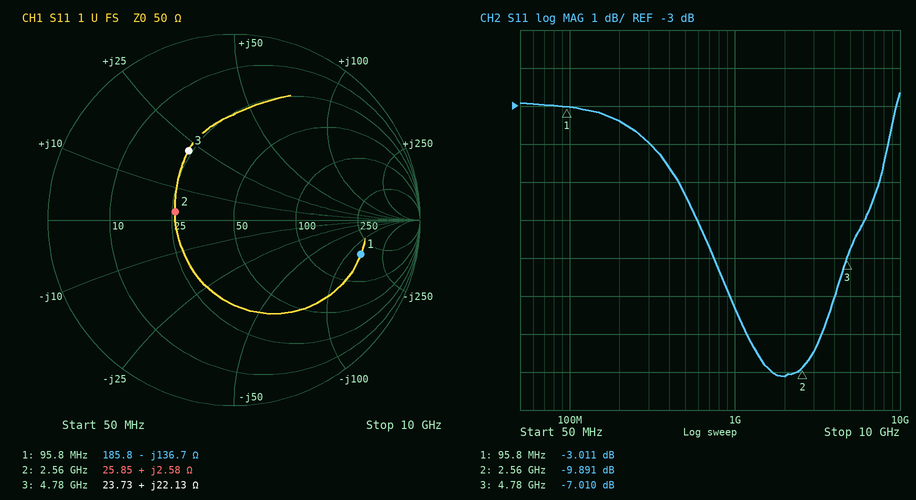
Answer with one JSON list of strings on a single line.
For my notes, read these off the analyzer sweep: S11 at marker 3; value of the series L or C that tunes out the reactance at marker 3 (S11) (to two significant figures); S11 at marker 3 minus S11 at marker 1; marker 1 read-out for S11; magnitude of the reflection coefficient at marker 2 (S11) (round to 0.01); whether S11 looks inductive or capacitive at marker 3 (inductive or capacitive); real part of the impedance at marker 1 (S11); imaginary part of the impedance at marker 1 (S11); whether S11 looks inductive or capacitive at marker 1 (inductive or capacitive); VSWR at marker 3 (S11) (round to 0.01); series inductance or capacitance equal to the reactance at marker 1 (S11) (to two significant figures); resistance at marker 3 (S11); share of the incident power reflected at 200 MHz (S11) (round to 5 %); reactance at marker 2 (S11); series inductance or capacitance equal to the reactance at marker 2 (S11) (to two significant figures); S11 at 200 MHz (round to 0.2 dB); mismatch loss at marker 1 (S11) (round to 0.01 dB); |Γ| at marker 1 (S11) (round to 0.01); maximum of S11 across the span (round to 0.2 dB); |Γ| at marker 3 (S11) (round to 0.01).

["-7.010 dB", "1.5 pF", "-3.999 dB", "-3.011 dB", "0.32", "inductive", "185.8 Ω", "-136.7 Ω", "capacitive", "2.61", "12 pF", "23.73 Ω", "45 %", "+2.58 Ω", "160 pH", "-3.4 dB", "3.01 dB", "0.71", "-2.6 dB", "0.45"]
